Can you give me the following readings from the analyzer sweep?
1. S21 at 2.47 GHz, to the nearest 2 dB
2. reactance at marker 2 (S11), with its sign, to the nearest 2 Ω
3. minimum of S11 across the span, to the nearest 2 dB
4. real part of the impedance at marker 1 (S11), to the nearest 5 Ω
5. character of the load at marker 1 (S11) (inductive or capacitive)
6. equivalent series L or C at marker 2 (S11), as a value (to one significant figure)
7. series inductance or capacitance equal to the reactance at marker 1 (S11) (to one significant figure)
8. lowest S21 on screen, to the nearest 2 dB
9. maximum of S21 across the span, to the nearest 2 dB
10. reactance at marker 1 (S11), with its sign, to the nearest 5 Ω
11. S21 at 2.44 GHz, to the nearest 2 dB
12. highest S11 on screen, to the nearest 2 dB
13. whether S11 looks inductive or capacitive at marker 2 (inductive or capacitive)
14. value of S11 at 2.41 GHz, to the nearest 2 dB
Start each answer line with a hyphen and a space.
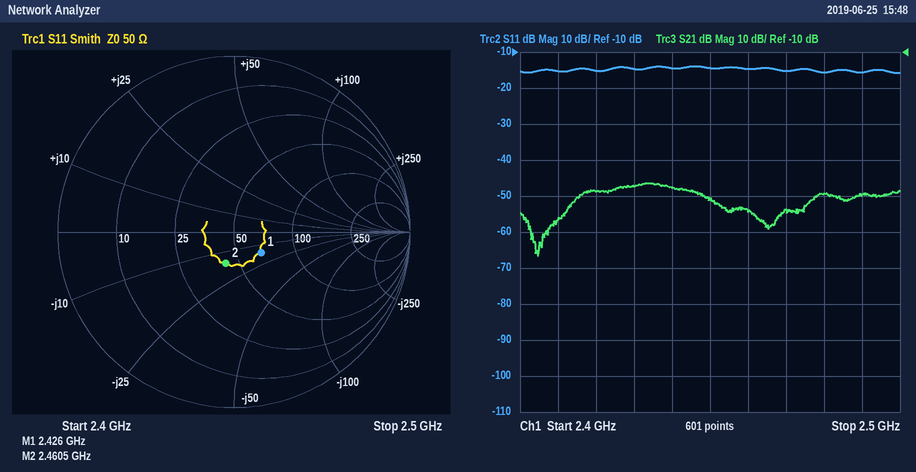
- -54 dB
- -16 Ω
- -16 dB
- 65 Ω
- capacitive
- 4 pF
- 4 pF
- -66 dB
- -46 dB
- -15 Ω
- -48 dB
- -14 dB
- capacitive
- -16 dB
